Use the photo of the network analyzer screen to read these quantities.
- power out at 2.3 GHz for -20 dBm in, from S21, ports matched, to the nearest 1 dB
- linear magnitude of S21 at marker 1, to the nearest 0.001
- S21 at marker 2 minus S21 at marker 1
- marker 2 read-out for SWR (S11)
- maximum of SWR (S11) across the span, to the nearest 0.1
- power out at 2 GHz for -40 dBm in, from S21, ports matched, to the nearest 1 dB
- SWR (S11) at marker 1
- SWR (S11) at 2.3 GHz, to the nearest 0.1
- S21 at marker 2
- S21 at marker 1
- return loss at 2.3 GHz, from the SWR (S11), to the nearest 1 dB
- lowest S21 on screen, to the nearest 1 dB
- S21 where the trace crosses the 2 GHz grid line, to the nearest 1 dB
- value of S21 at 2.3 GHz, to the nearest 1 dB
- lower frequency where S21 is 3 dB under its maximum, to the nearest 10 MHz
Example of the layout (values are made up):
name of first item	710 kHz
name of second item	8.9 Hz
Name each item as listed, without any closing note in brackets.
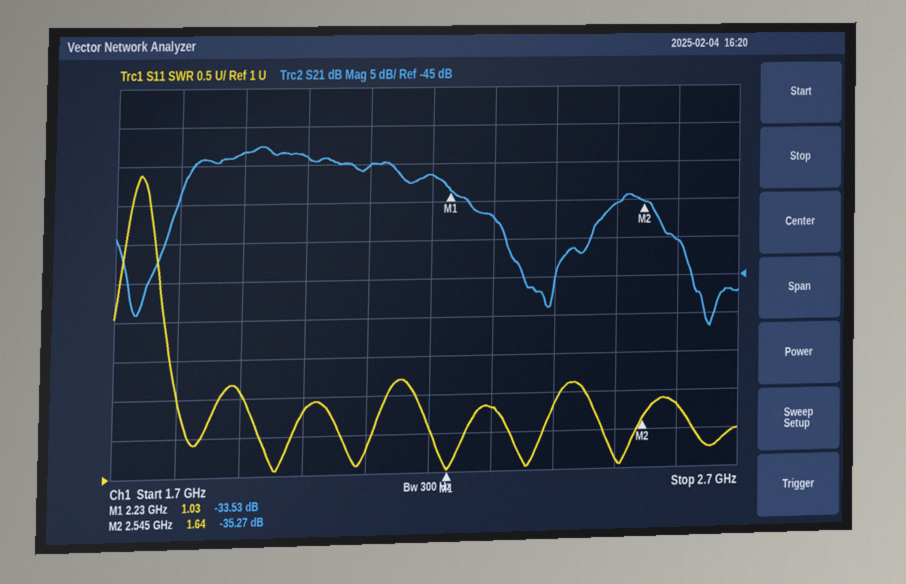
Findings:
power out at 2.3 GHz for -20 dBm in, from S21, ports matched, to the nearest 1 dB	-57 dBm
linear magnitude of S21 at marker 1, to the nearest 0.001	0.021
S21 at marker 2 minus S21 at marker 1	-1.74 dB
marker 2 read-out for SWR	1.64
maximum of SWR (S11) across the span, to the nearest 0.1	4.9
power out at 2 GHz for -40 dBm in, from S21, ports matched, to the nearest 1 dB	-69 dBm
SWR (S11) at marker 1	1.03
SWR (S11) at 2.3 GHz, to the nearest 0.1	1.8
S21 at marker 2	-35.27 dB
S21 at marker 1	-33.53 dB
return loss at 2.3 GHz, from the SWR (S11), to the nearest 1 dB	11 dB
lowest S21 on screen, to the nearest 1 dB	-52 dB
S21 where the trace crosses the 2 GHz grid line, to the nearest 1 dB	-29 dB
value of S21 at 2.3 GHz, to the nearest 1 dB	-37 dB
lower frequency where S21 is 3 dB under its maximum, to the nearest 10 MHz	1.82 GHz
